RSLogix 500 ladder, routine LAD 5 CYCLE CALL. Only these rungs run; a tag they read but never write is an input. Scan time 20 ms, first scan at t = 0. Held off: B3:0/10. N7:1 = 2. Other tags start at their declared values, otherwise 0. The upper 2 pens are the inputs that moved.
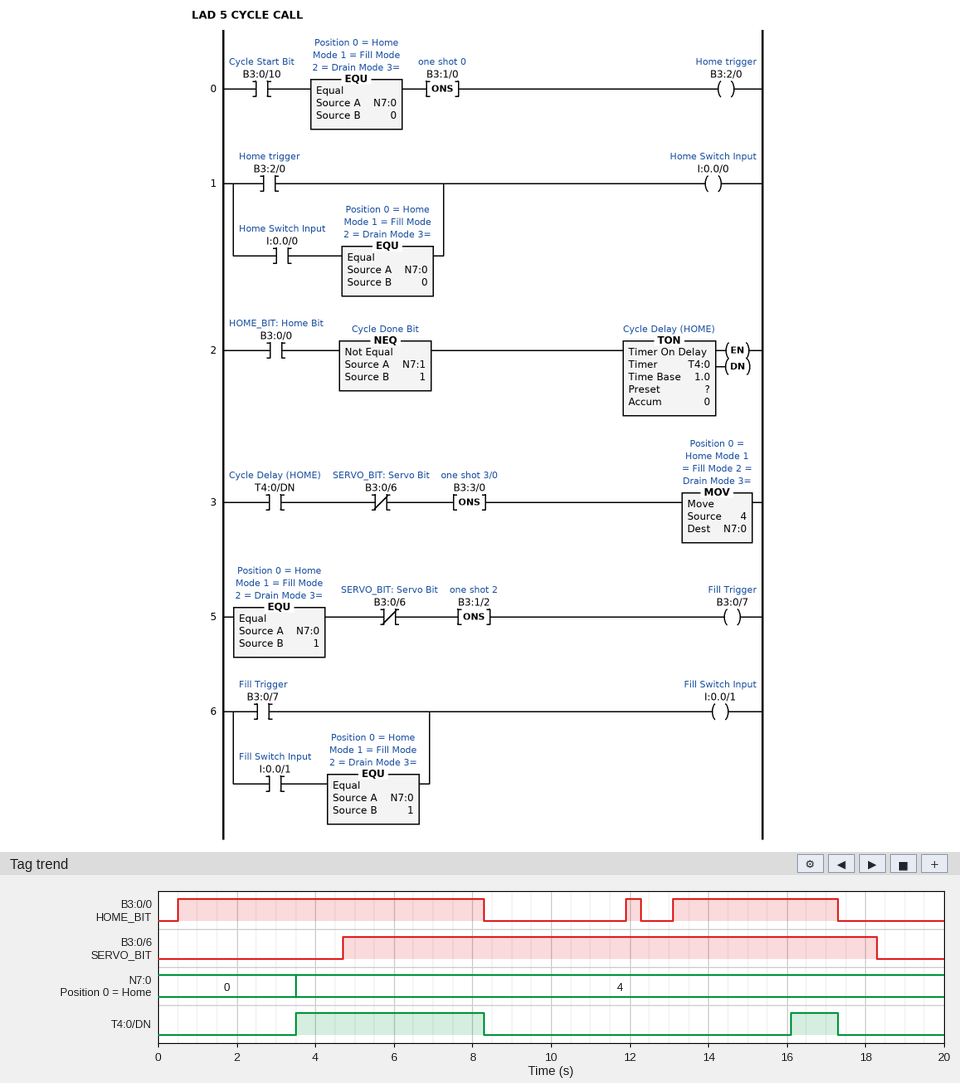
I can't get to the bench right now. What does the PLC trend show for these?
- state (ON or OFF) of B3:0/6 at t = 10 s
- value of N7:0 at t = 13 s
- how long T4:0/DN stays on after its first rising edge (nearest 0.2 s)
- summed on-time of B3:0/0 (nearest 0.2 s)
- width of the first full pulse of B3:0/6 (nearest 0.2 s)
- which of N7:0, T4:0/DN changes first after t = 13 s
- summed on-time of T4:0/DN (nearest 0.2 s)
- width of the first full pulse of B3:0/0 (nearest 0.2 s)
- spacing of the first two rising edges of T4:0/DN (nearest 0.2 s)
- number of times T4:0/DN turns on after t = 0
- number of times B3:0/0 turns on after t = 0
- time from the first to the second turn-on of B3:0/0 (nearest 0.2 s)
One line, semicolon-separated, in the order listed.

ON; 4; 4.8 s; 12.4 s; 13.6 s; T4:0/DN; 6.0 s; 7.8 s; 12.6 s; 2; 3; 11.4 s
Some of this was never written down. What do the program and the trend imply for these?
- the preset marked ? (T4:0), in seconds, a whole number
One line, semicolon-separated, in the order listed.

3 s
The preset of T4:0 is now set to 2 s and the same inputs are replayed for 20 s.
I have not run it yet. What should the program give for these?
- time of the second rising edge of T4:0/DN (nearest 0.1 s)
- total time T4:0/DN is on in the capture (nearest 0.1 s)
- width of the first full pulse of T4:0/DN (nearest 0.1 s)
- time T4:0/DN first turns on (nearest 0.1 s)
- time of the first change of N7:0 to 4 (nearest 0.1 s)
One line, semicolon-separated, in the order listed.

15.1 s; 8.0 s; 5.8 s; 2.5 s; 2.5 s
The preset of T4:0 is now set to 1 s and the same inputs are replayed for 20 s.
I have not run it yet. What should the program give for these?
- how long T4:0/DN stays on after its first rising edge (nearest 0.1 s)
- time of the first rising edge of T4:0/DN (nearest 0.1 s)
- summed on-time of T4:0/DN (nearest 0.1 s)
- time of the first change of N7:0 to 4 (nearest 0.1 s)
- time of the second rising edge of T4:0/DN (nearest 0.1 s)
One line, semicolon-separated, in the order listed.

6.8 s; 1.5 s; 10.0 s; 1.5 s; 14.1 s
